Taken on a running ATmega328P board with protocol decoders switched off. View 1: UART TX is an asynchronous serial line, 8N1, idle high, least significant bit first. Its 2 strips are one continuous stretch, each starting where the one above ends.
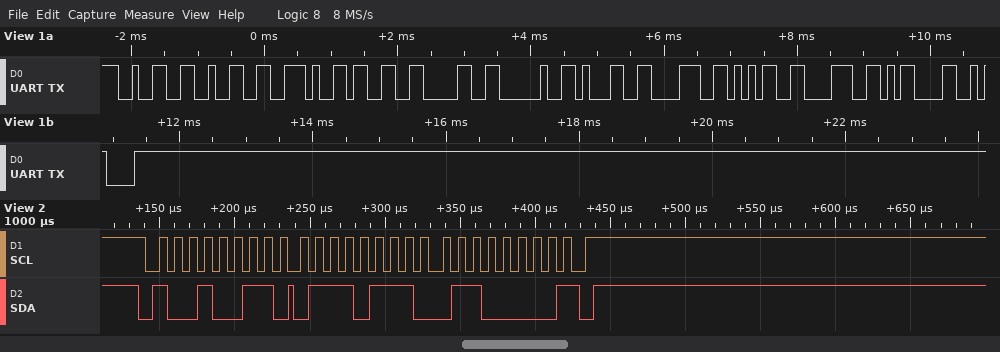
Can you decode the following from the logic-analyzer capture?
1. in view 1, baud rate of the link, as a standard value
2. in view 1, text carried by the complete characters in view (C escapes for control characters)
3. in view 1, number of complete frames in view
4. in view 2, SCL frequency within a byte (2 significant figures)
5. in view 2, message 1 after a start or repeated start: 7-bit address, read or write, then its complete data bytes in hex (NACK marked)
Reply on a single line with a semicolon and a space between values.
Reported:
9600 baud; "22.30 1858\r\n"; 12; 100 kHz; 0x49 read: 77 60 NACK
